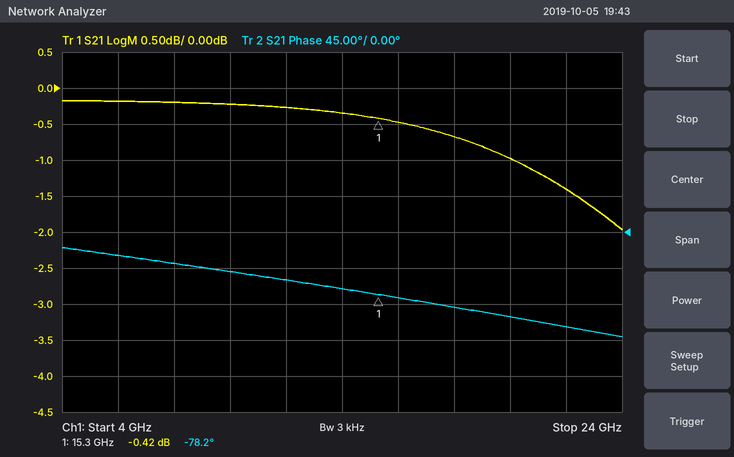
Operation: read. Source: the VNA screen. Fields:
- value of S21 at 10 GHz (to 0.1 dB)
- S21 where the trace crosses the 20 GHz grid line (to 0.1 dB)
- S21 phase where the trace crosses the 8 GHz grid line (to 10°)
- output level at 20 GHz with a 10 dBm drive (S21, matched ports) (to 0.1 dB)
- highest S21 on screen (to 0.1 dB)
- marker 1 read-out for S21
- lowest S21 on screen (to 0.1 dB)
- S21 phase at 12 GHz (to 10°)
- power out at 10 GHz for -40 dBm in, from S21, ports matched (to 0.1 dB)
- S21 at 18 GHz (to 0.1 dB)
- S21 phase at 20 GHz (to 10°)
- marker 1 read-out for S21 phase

-0.2 dB
-1.0 dB
-40°
9.0 dBm
-0.2 dB
-0.42 dB
-2.0 dB
-60°
-40.2 dBm
-0.7 dB
-110°
-78.2°
